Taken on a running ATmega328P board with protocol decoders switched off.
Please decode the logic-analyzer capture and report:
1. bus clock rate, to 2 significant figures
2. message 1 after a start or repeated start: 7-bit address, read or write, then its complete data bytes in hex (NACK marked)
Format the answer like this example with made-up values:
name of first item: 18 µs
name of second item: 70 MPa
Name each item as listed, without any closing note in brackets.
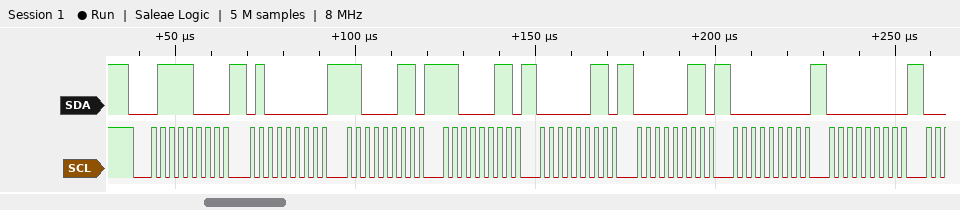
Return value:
bus clock rate, to 2 significant figures: 400 kHz
message 1 after a start or repeated start: 7-bit address, read or write, then its complete data bytes in hex: 0x3C write: 40 C3 C3 03 03 00 00
